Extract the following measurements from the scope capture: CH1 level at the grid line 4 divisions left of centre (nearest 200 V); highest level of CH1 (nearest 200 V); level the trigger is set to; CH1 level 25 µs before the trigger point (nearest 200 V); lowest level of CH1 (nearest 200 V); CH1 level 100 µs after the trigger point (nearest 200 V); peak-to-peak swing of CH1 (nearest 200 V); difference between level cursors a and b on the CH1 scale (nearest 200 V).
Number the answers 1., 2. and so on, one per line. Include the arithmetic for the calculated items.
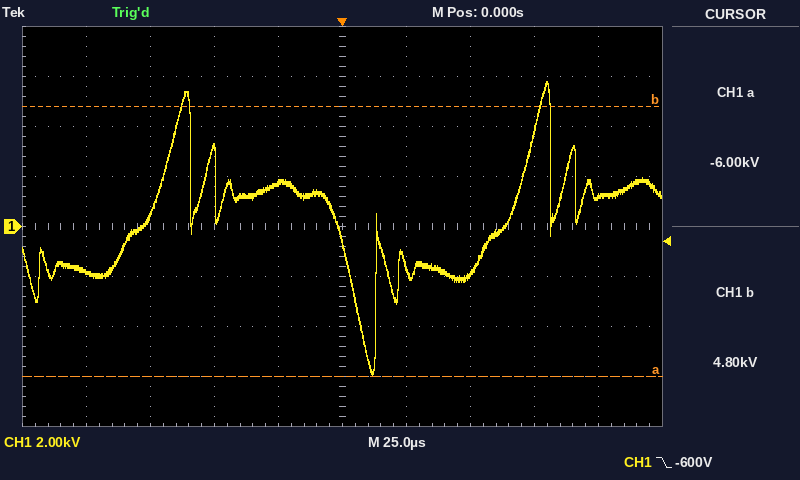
1. -1.8 kV
2. 5.8 kV
3. -600 V
4. 1.8 kV
5. -6.0 kV
6. 1.2 kV
7. 5.8 kV − (-6.0 kV) = 11.8 kV
8. 10.8 kV
